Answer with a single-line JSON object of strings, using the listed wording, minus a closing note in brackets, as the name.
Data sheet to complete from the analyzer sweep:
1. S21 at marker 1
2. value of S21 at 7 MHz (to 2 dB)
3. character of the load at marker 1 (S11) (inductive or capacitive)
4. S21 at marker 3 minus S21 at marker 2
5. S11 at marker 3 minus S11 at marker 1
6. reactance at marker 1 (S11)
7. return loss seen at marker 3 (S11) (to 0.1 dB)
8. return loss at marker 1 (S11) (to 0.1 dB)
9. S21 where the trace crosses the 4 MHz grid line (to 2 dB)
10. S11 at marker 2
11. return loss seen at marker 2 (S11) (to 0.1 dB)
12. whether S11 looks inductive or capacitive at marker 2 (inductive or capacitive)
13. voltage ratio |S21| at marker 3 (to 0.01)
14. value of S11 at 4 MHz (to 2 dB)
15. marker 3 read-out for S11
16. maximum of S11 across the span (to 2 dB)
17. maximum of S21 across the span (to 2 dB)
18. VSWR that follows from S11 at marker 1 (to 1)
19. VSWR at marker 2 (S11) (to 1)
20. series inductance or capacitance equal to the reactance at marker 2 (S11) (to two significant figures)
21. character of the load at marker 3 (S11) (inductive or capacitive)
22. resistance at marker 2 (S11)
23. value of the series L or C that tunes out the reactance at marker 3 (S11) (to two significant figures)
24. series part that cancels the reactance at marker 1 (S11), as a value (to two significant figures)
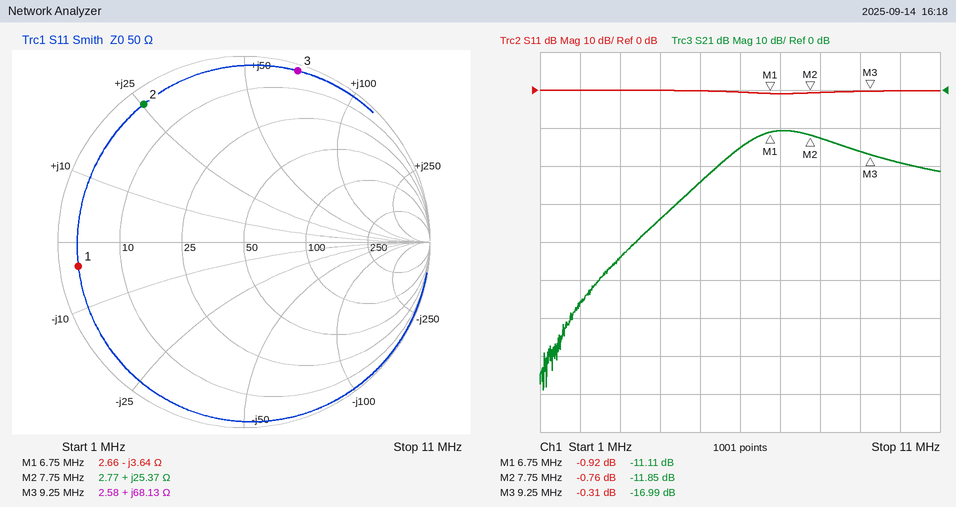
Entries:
{"S21 at marker 1": "-11.11 dB", "value of S21 at 7 MHz": "-10 dB", "character of the load at marker 1 (S11)": "capacitive", "S21 at marker 3 minus S21 at marker 2": "-5.14 dB", "S11 at marker 3 minus S11 at marker 1": "0.61 dB", "reactance at marker 1": "-3.64 Ω", "return loss seen at marker 3 (S11)": "0.3 dB", "return loss at marker 1 (S11)": "0.9 dB", "S21 where the trace crosses the 4 MHz grid line": "-34 dB", "S11 at marker 2": "-0.76 dB", "return loss seen at marker 2 (S11)": "0.8 dB", "whether S11 looks inductive or capacitive at marker 2": "inductive", "voltage ratio |S21| at marker 3": "0.14", "value of S11 at 4 MHz": "0 dB", "marker 3 read-out for S11": "-0.31 dB", "maximum of S11 across the span": "0 dB", "maximum of S21 across the span": "-10 dB", "VSWR that follows from S11 at marker 1": "19", "VSWR at marker 2 (S11)": "23", "series inductance or capacitance equal to the reactance at marker 2 (S11)": "520 nH", "character of the load at marker 3 (S11)": "inductive", "resistance at marker 2": "2.77 Ω", "value of the series L or C that tunes out the reactance at marker 3 (S11)": "250 pF", "series part that cancels the reactance at marker 1 (S11), as a value": "86 nH"}
